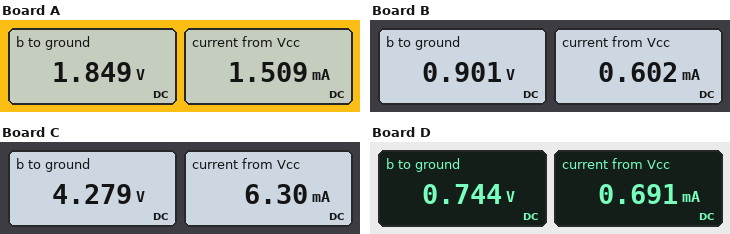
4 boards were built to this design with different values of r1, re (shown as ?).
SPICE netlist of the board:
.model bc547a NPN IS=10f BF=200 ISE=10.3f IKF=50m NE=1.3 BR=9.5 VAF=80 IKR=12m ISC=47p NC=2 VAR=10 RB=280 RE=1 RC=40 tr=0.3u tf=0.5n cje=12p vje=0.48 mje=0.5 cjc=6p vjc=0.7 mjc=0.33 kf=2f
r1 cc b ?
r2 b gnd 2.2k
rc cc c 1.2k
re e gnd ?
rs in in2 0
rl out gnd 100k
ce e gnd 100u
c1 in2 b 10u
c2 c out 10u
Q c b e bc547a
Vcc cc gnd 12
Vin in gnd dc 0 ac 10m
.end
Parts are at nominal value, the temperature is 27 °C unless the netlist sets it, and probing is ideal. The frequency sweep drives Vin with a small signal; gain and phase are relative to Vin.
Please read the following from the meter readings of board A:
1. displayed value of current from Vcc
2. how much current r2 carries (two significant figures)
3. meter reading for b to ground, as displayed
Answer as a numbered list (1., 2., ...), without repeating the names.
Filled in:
1. 1.509 mA
2. 840 µA
3. 1.849 V
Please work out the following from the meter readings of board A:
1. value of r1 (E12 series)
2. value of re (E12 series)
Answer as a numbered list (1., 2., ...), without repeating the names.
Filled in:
1. 12 kΩ
2. 1.8 kΩ
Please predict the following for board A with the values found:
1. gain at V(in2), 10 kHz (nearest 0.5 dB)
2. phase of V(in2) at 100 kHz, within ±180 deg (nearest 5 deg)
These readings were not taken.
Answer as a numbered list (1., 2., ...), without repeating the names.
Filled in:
1. 0 dB
2. 0 deg
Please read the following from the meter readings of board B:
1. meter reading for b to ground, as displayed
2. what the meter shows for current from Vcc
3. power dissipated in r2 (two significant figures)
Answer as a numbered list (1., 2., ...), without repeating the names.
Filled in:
1. 0.901 V
2. 0.602 mA
3. 370 µW
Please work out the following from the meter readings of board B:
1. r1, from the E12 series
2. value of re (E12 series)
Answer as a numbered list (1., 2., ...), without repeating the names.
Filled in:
1. 27 kΩ
2. 1.5 kΩ
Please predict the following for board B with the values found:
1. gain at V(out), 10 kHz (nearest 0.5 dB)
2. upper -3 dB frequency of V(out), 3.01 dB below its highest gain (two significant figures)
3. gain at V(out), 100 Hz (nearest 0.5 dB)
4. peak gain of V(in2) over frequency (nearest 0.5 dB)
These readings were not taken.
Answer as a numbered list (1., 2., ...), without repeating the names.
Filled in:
1. 18.5 dB
2. 9.2 MHz
3. 18.5 dB
4. 0 dB
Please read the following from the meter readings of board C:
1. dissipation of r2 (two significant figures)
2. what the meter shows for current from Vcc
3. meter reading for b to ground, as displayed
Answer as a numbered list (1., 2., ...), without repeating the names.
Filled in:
1. 8.3 mW
2. 6.30 mA
3. 4.279 V
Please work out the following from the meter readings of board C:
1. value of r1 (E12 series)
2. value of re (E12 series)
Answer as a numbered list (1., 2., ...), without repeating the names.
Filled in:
1. 3.9 kΩ
2. 820 Ω
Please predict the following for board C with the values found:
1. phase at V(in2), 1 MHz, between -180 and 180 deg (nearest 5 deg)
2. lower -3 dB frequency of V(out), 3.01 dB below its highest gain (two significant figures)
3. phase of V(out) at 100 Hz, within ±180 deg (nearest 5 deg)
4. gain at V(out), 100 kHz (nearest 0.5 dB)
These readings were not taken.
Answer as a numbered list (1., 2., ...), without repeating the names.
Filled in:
1. 0 deg
2. 170 Hz
3. -115 deg
4. 41.0 dB
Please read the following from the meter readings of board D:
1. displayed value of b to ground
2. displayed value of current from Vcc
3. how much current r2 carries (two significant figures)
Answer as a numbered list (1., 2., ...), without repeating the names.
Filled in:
1. 0.744 V
2. 0.691 mA
3. 340 µA
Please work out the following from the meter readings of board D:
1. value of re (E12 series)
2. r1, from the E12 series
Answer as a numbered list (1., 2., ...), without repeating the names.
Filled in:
1. 330 Ω
2. 33 kΩ
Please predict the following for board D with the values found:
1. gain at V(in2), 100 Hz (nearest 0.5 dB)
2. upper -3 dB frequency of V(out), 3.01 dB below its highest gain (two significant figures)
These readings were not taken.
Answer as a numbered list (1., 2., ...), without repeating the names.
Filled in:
1. 0 dB
2. 7.0 MHz
